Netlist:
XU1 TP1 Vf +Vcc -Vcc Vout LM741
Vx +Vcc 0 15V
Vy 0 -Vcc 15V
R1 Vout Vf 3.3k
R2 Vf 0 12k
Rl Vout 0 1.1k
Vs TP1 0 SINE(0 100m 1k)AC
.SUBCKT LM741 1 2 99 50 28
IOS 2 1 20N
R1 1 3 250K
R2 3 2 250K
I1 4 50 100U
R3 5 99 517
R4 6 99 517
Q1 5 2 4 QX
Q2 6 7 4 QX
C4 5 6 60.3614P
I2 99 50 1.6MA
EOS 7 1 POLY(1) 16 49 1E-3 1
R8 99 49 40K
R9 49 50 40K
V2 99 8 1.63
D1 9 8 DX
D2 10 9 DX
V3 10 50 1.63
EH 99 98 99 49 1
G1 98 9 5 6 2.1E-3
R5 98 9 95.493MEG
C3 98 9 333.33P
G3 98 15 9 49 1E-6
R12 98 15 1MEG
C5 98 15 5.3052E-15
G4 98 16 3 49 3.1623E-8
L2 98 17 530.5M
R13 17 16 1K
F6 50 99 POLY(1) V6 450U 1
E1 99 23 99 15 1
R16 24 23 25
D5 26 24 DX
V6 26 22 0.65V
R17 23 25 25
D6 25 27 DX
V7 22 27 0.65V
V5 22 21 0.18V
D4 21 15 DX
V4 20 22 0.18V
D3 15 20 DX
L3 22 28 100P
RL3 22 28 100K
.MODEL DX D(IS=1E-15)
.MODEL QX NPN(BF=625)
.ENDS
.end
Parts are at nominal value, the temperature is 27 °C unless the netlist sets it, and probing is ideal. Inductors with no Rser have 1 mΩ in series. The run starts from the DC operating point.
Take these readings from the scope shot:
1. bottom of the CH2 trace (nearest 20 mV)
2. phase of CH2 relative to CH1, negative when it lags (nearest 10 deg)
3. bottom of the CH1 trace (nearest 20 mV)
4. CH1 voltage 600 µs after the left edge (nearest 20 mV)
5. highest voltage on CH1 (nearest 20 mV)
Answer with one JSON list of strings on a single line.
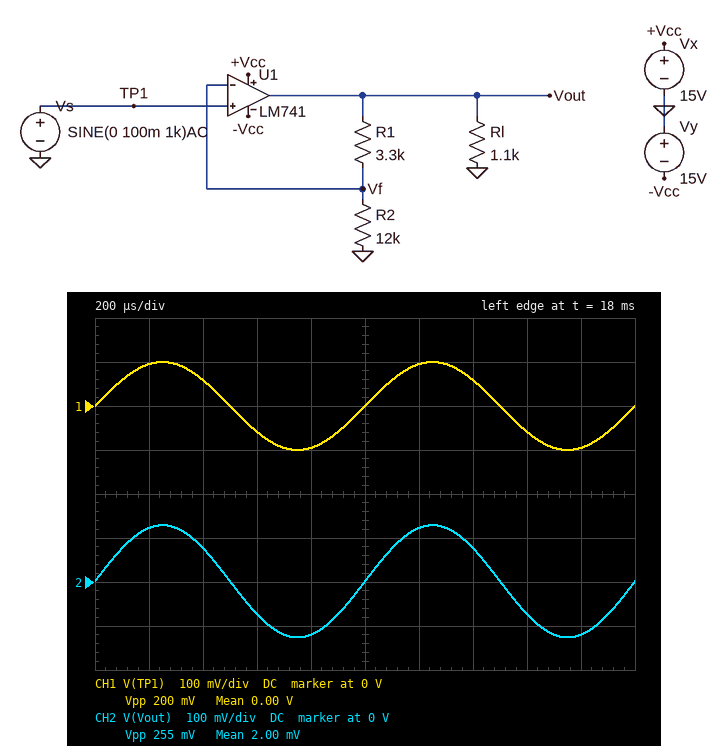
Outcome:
["-120 mV", "0 deg", "-100 mV", "-60 mV", "100 mV"]
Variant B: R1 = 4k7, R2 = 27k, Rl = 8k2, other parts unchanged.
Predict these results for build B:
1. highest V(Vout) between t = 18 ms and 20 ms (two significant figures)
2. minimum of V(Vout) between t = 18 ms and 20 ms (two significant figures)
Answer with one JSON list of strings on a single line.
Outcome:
["120 mV", "-120 mV"]
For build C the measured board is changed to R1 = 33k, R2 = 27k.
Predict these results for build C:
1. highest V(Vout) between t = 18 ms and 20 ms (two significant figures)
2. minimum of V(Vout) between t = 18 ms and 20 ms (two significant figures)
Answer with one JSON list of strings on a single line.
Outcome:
["230 mV", "-220 mV"]
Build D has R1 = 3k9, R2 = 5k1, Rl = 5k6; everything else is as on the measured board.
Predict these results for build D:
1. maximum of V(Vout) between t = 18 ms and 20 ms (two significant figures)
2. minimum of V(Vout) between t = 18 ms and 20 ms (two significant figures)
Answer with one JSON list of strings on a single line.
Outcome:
["180 mV", "-170 mV"]
